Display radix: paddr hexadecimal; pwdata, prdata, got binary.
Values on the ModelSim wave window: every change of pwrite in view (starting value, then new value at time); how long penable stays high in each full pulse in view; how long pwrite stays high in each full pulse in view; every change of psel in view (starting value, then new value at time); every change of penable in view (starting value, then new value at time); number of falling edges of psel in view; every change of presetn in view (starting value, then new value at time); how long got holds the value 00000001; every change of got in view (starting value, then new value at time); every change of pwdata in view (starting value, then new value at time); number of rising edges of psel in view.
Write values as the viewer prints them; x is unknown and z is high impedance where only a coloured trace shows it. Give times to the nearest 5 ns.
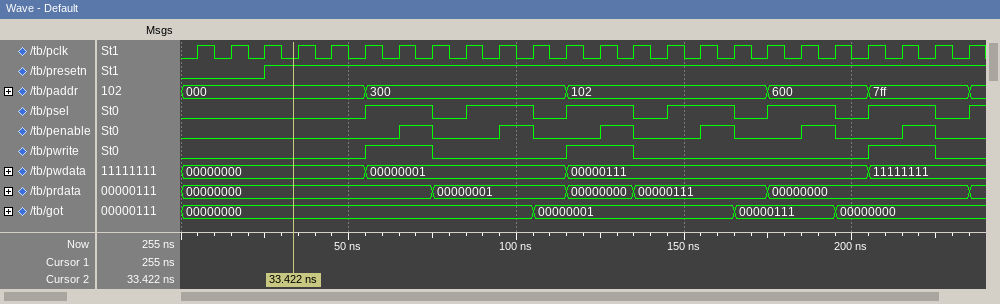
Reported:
0, 1 at 55 ns, 0 at 75 ns, 1 at 115 ns, 0 at 135 ns, 1 at 205 ns, 0 at 225 ns
10 ns, 10 ns, 10 ns, 10 ns, 10 ns, 10 ns
20 ns, 20 ns, 20 ns
0, 1 at 55 ns, 0 at 75 ns, 1 at 85 ns, 0 at 105 ns, 1 at 115 ns, 0 at 135 ns, 1 at 145 ns, 0 at 165 ns, 1 at 175 ns, 0 at 195 ns, 1 at 205 ns, 0 at 225 ns, 1 at 235 ns
0, 1 at 65 ns, 0 at 75 ns, 1 at 95 ns, 0 at 105 ns, 1 at 125 ns, 0 at 135 ns, 1 at 155 ns, 0 at 165 ns, 1 at 185 ns, 0 at 195 ns, 1 at 215 ns, 0 at 225 ns
6
0, 1 at 25 ns
60 ns
00000000, 00000001 at 105 ns, 00000111 at 165 ns, 00000000 at 195 ns
00000000, 00000001 at 55 ns, 00000111 at 115 ns, 11111111 at 205 ns
7
